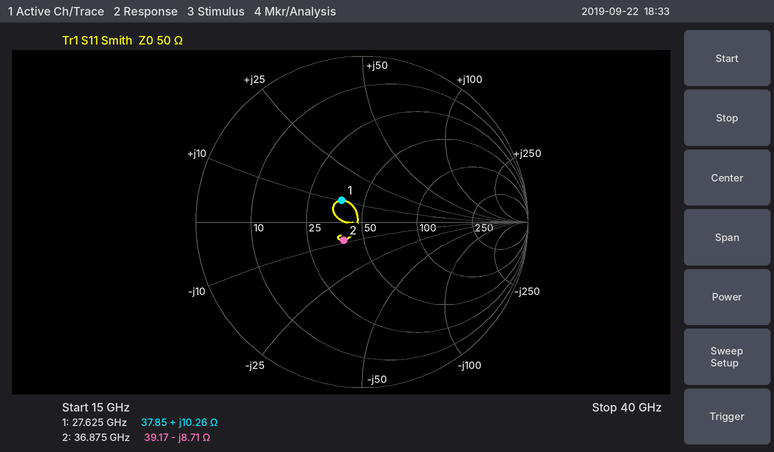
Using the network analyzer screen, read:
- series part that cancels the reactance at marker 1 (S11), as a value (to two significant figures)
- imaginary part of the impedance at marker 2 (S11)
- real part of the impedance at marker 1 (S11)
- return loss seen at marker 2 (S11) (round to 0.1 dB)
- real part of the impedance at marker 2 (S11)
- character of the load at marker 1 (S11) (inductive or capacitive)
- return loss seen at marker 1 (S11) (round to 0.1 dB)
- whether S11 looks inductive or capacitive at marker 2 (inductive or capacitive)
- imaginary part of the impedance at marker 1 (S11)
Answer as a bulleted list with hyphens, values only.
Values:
- 560 fF
- -8.71 Ω
- 37.85 Ω
- 16.2 dB
- 39.17 Ω
- inductive
- 14.9 dB
- capacitive
- +10.26 Ω
